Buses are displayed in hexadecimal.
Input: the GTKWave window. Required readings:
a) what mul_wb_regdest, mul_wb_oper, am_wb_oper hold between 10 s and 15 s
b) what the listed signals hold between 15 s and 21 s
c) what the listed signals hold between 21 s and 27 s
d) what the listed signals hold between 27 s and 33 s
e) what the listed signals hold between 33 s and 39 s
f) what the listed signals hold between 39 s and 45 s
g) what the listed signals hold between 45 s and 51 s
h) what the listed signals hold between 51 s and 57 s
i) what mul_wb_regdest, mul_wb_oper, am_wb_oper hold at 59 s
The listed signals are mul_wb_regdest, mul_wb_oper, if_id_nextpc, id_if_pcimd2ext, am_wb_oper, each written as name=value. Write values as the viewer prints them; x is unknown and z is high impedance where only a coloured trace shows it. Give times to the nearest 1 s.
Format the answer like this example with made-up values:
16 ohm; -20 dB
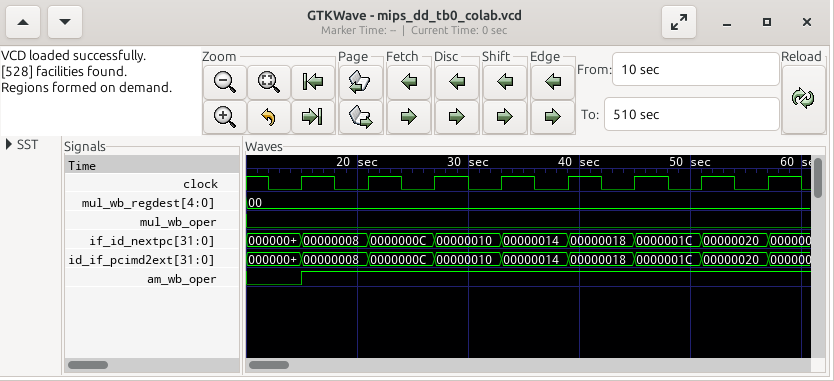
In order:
mul_wb_regdest=00, mul_wb_oper=0, am_wb_oper=0; mul_wb_regdest=00, mul_wb_oper=0, if_id_nextpc=00000008, id_if_pcimd2ext=00000008, am_wb_oper=1; mul_wb_regdest=00, mul_wb_oper=0, if_id_nextpc=0000000C, id_if_pcimd2ext=0000000C, am_wb_oper=1; mul_wb_regdest=00, mul_wb_oper=0, if_id_nextpc=00000010, id_if_pcimd2ext=00000010, am_wb_oper=1; mul_wb_regdest=00, mul_wb_oper=0, if_id_nextpc=00000014, id_if_pcimd2ext=00000014, am_wb_oper=1; mul_wb_regdest=00, mul_wb_oper=0, if_id_nextpc=00000018, id_if_pcimd2ext=00000018, am_wb_oper=1; mul_wb_regdest=00, mul_wb_oper=0, if_id_nextpc=0000001C, id_if_pcimd2ext=0000001C, am_wb_oper=1; mul_wb_regdest=00, mul_wb_oper=0, if_id_nextpc=00000020, id_if_pcimd2ext=00000020, am_wb_oper=1; mul_wb_regdest=00, mul_wb_oper=0, am_wb_oper=1
